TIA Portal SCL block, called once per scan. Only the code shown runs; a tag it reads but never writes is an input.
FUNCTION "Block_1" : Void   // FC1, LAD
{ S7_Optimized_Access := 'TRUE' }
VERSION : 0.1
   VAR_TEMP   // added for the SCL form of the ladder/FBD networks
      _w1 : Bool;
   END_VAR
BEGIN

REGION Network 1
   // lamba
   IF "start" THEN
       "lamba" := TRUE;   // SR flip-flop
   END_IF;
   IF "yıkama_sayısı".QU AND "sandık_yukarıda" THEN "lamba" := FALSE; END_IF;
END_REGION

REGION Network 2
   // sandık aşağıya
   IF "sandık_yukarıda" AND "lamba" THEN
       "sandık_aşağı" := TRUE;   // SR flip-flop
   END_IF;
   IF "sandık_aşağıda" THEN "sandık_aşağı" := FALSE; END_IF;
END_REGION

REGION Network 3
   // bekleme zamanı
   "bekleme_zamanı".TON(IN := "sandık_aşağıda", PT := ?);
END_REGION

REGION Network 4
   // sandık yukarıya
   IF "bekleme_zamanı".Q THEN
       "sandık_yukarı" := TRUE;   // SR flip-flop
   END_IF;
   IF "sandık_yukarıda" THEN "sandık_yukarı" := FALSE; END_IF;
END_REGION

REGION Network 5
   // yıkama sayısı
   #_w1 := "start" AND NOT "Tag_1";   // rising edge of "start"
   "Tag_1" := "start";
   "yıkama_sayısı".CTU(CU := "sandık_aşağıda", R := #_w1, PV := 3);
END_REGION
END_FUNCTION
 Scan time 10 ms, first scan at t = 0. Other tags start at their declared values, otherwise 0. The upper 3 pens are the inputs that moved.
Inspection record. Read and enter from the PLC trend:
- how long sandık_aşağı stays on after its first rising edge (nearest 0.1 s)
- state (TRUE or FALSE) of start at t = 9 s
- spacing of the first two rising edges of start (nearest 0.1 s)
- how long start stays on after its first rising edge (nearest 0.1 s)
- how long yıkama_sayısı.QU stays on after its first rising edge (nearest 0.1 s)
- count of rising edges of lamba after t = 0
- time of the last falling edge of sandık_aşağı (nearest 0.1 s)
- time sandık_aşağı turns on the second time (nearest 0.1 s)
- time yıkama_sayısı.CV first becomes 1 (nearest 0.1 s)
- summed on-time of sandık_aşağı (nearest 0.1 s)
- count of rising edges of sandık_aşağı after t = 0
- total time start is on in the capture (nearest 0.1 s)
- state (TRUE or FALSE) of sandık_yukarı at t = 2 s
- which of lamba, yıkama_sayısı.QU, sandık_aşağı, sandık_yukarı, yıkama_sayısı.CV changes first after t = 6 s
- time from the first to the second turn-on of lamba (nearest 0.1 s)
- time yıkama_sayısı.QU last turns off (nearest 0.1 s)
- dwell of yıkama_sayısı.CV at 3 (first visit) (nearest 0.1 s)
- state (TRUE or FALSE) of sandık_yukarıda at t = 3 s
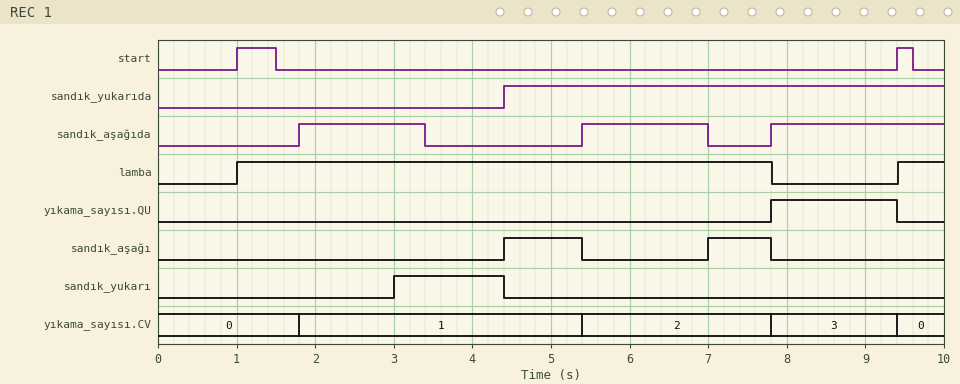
1.0 s
FALSE
8.4 s
0.5 s
1.6 s
2
7.8 s
7.0 s
1.8 s
1.8 s
2
0.7 s
FALSE
sandık_aşağı
8.4 s
9.4 s
1.6 s
FALSE
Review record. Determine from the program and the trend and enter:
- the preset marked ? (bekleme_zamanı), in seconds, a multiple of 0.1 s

1.2 s
